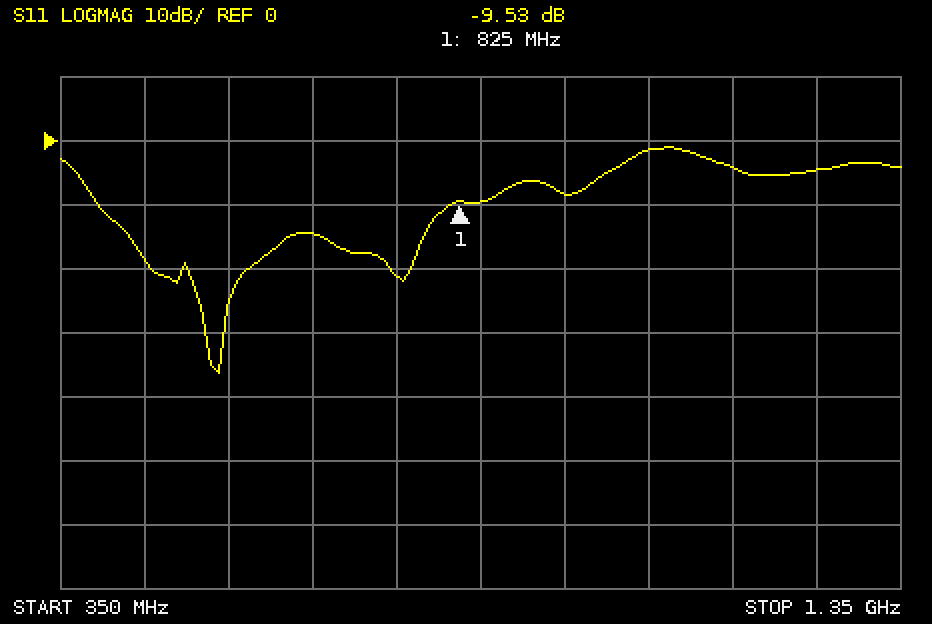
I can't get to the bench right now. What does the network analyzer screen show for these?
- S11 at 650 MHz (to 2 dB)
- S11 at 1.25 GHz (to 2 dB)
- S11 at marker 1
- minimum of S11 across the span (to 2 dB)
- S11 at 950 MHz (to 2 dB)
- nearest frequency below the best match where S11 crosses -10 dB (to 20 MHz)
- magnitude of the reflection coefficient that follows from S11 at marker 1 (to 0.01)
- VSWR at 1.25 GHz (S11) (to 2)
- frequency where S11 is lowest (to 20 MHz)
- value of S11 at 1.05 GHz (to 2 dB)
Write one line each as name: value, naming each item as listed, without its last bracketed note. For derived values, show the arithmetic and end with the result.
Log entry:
S11 at 650 MHz: -14 dB
S11 at 1.25 GHz: -4 dB
S11 at marker 1: -9.53 dB
minimum of S11 across the span: -36 dB
S11 at 950 MHz: -8 dB
nearest frequency below the best match where S11 crosses -10 dB: 400 MHz
magnitude of the reflection coefficient that follows from S11 at marker 1: 10^(-9.53/20) ≈ 0.33
VSWR at 1.25 GHz (S11): |Γ| = 10^(-4/20) = 0.6310; VSWR = (1 + 0.6310)/(1 − 0.6310) ≈ 4
frequency where S11 is lowest: 540 MHz
value of S11 at 1.05 GHz: -2 dB
